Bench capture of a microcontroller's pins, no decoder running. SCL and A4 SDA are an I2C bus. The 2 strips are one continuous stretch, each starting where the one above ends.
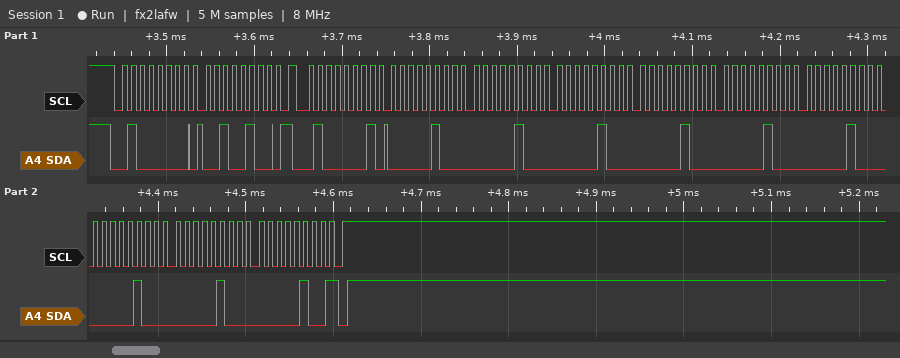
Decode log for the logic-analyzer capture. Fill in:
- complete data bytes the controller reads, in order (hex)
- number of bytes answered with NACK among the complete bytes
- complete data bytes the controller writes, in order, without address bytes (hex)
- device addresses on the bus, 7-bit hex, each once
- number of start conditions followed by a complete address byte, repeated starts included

04 04 04 04 04 04 04 04 04
1
24
0x20
2
